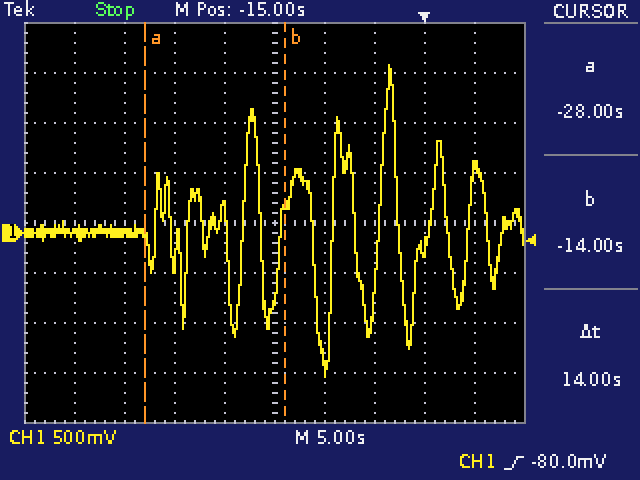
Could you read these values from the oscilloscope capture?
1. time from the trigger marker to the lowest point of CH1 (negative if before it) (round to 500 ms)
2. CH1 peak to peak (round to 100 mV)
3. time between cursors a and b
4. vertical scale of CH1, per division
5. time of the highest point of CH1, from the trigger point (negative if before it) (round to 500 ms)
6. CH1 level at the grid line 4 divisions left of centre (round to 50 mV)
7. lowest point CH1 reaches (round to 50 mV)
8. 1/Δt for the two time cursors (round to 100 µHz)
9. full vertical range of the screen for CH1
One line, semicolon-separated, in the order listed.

-10.0 s; 3.10 V; 14 s; 500 mV; -3.5 s; 0 mV; -1.45 V; 71.4 mHz; 4 V
